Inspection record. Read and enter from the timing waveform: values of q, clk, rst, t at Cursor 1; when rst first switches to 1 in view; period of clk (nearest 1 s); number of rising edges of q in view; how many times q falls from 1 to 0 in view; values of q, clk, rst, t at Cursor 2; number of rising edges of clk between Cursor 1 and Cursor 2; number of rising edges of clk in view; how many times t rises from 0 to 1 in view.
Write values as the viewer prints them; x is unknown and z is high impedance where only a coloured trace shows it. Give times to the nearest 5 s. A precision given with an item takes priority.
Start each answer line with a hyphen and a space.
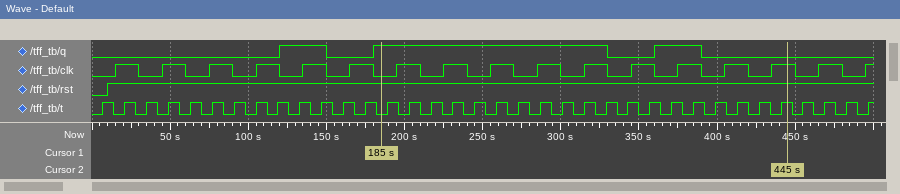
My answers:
- q=1, clk=0, rst=1, t=0
- 10 s
- 30 s
- 3
- 3
- q=0, clk=1, rst=1, t=1
- 9
- 17
- 36
